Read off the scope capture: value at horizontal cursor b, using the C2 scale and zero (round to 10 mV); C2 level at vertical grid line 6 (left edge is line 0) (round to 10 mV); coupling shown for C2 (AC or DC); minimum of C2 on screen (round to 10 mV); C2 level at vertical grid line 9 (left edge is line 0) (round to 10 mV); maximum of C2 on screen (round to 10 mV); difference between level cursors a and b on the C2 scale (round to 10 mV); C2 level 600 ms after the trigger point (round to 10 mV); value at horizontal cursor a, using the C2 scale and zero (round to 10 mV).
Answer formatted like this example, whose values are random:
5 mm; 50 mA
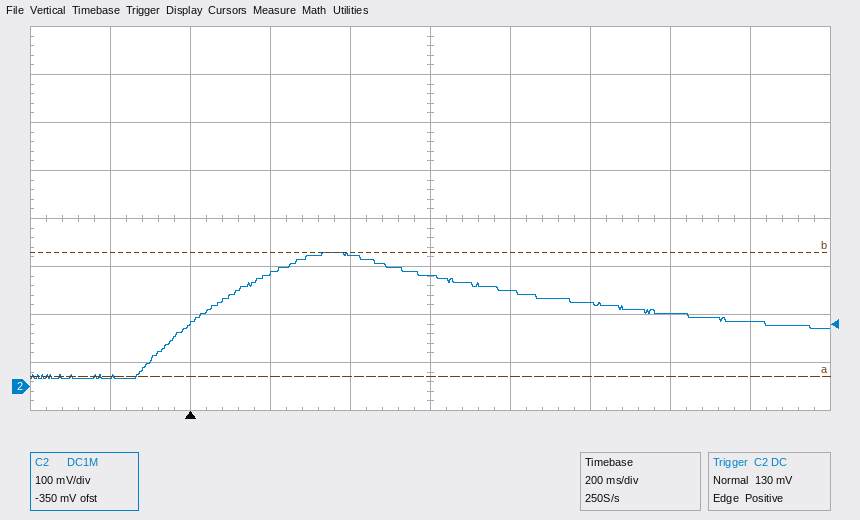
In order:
280 mV; 200 mV; DC; 20 mV; 140 mV; 280 mV; 260 mV; 230 mV; 20 mV
